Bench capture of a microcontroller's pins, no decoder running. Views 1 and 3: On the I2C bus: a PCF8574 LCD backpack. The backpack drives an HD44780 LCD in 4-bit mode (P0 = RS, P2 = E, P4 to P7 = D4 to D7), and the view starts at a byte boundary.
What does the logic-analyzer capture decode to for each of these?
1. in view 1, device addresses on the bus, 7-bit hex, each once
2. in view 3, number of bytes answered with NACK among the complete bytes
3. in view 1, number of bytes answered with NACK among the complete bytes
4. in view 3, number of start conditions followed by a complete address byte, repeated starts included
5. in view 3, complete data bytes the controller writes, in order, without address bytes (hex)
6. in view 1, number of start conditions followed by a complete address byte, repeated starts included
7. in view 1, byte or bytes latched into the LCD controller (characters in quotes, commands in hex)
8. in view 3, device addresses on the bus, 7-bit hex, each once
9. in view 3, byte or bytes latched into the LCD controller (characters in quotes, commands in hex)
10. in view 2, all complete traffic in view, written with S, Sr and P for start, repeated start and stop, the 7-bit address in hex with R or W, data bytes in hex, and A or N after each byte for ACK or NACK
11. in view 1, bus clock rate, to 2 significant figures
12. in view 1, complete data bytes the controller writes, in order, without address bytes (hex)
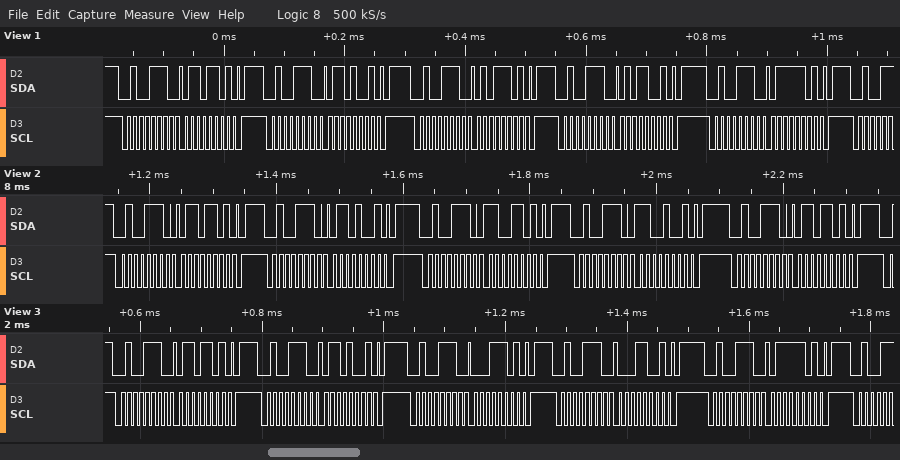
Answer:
0x27
0
0
5
6D 69 1D 19 7D
5
'e'
0x27
'a'
S 27W A 6D A P S 27W A 69 A P S 27W A CD A P S 27W A C9 A P S 27W A 6D A P
100 kHz
6D 69 5D 59 7D
